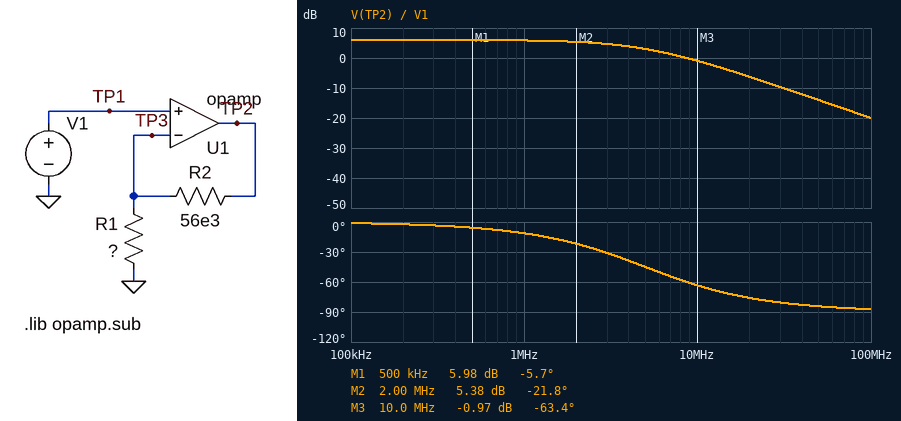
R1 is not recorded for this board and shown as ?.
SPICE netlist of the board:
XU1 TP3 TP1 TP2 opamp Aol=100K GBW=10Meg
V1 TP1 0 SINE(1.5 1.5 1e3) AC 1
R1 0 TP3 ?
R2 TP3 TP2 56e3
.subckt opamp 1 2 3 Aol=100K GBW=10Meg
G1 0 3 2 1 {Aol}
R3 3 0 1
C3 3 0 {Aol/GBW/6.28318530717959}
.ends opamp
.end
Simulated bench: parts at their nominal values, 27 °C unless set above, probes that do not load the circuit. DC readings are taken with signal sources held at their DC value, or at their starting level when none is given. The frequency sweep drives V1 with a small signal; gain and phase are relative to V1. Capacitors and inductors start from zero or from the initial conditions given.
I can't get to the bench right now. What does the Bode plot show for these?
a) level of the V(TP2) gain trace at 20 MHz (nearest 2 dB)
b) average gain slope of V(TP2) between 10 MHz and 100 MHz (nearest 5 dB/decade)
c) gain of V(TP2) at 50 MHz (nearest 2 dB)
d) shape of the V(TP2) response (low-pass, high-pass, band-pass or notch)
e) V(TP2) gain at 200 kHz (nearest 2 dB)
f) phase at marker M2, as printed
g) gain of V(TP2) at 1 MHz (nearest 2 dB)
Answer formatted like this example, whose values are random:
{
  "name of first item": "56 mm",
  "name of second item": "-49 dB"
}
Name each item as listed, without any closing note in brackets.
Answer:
{
  "level of the V(TP2) gain trace at 20 MHz": "-6 dB",
  "average gain slope of V(TP2) between 10 MHz and 100 MHz": "-20 dB/decade",
  "gain of V(TP2) at 50 MHz": "-14 dB",
  "shape of the V(TP2) response": "low-pass",
  "V(TP2) gain at 200 kHz": "6 dB",
  "phase at marker M2, as printed": "-21.8 deg",
  "gain of V(TP2) at 1 MHz": "6 dB"
}
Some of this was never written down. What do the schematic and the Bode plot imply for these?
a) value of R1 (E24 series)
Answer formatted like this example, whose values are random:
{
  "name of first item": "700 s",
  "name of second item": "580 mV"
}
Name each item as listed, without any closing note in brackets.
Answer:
{
  "value of R1": "56 kΩ"
}
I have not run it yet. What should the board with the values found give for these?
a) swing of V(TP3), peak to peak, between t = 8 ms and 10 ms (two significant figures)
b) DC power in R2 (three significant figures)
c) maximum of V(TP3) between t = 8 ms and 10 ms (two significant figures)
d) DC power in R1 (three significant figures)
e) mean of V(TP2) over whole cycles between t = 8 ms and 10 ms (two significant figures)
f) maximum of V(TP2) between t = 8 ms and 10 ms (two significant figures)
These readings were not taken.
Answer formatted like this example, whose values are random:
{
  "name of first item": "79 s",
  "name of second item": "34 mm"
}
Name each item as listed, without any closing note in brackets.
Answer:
{
  "swing of V(TP3), peak to peak, between t = 8 ms and 10 ms": "3.0 V",
  "DC power in R2": "40.2 µW",
  "maximum of V(TP3) between t = 8 ms and 10 ms": "3.0 V",
  "DC power in R1": "40.2 µW",
  "mean of V(TP2) over whole cycles between t = 8 ms and 10 ms": "3.0 V",
  "maximum of V(TP2) between t = 8 ms and 10 ms": "6.0 V"
}
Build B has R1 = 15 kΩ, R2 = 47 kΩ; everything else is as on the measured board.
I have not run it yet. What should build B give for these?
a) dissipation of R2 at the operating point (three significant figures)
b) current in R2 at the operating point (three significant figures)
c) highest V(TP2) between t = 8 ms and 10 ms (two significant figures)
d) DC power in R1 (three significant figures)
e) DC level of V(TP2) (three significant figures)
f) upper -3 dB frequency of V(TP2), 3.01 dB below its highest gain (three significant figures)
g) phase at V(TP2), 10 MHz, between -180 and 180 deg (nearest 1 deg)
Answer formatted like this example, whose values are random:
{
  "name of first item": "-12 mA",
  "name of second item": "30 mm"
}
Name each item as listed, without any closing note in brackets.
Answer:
{
  "dissipation of R2 at the operating point": "470 µW",
  "current in R2 at the operating point": "100 µA",
  "highest V(TP2) between t = 8 ms and 10 ms": "12 V",
  "DC power in R1": "150 µW",
  "DC level of V(TP2)": "6.20 V",
  "upper -3 dB frequency of V(TP2), 3.01 dB below its highest gain": "2.42 MHz",
  "phase at V(TP2), 10 MHz, between -180 and 180 deg": "-76 deg"
}
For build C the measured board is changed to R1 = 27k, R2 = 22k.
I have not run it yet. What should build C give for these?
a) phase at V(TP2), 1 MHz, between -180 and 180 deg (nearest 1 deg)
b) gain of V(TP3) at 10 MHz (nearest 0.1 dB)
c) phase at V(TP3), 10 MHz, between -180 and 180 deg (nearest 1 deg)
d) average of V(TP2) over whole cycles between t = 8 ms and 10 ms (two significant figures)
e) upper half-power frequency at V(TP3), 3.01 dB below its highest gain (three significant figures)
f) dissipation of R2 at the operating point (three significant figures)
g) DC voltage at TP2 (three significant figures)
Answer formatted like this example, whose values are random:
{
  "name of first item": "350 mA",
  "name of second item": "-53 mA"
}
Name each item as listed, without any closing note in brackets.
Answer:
{
  "phase at V(TP2), 1 MHz, between -180 and 180 deg": "-10 deg",
  "gain of V(TP3) at 10 MHz": "-6.3 dB",
  "phase at V(TP3), 10 MHz, between -180 and 180 deg": "-61 deg",
  "average of V(TP2) over whole cycles between t = 8 ms and 10 ms": "2.7 V",
  "upper half-power frequency at V(TP3), 3.01 dB below its highest gain": "5.51 MHz",
  "dissipation of R2 at the operating point": "67.9 µW",
  "DC voltage at TP2": "2.72 V"
}
